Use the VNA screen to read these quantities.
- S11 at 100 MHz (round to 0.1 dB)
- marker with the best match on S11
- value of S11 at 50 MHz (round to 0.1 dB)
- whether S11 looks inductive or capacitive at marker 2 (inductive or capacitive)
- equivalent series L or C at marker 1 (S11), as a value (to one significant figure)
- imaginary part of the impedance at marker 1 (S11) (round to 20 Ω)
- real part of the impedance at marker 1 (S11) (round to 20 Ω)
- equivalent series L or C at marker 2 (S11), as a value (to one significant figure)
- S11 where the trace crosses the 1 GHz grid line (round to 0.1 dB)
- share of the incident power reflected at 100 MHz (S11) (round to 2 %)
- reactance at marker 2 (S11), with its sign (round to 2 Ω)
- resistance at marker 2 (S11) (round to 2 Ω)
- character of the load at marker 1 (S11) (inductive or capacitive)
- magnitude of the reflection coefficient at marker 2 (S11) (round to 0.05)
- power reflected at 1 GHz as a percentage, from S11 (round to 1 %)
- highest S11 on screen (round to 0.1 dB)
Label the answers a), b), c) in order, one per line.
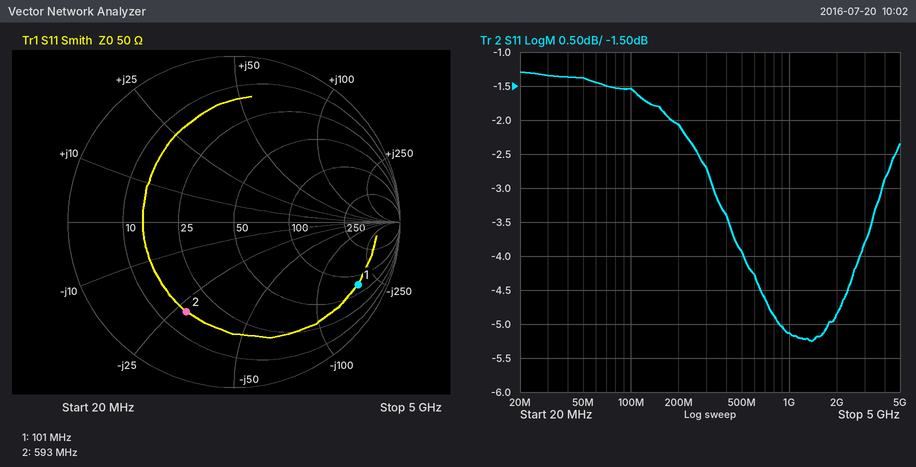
a) -1.5 dB
b) marker 2
c) -1.4 dB
d) capacitive
e) 9 pF
f) -180 Ω
g) 80 Ω
h) 10 pF
i) -5.1 dB
j) 70 %
k) -28 Ω
l) 16 Ω
m) capacitive
n) 0.60
o) 31 %
p) -1.3 dB
